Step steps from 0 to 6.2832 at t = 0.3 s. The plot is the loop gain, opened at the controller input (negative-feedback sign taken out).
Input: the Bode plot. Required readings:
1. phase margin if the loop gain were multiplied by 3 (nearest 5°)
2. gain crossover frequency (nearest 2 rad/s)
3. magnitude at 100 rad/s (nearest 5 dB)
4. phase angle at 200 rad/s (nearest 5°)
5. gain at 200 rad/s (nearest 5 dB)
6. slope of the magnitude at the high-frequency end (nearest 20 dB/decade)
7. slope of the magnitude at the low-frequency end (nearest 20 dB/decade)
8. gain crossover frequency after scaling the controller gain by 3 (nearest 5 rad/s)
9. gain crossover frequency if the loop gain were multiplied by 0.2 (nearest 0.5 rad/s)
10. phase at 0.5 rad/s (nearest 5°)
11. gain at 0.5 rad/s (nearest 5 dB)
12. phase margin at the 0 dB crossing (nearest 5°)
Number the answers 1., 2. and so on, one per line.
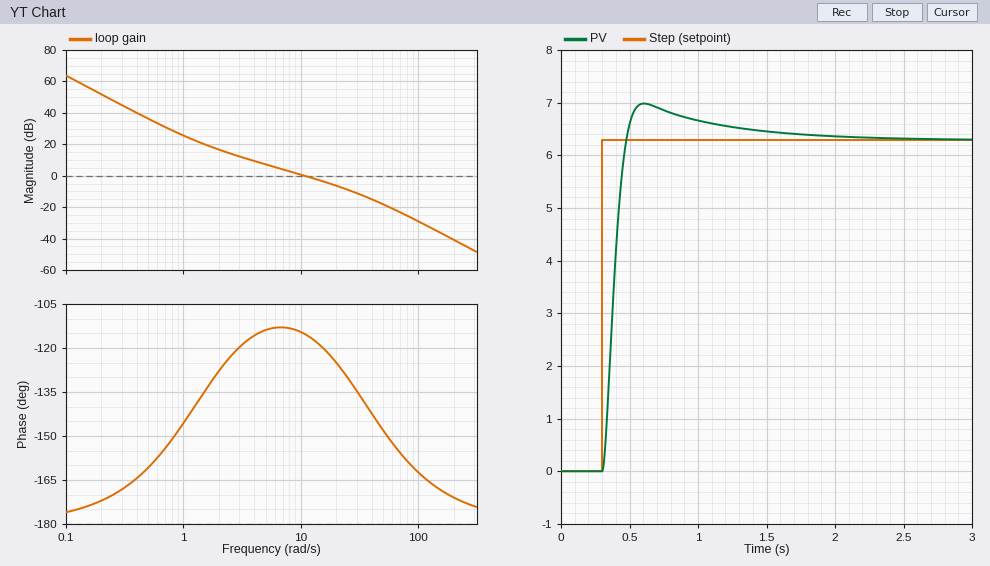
1. 50°
2. 10 rad/s
3. -30 dB
4. -170°
5. -40 dB
6. -40 dB/decade
7. -40 dB/decade
8. 25 rad/s
9. 2.5 rad/s
10. -160°
11. 35 dB
12. 65°
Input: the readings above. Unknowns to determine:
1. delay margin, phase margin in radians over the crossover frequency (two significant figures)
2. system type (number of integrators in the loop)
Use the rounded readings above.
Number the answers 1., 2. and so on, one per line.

1. 0.11 s
2. 2
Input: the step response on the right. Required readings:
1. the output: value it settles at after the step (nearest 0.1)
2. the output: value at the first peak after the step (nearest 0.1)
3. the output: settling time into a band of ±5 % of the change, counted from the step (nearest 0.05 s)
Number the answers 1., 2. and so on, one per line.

1. 6.3
2. 7.0
3. 0.80 s
